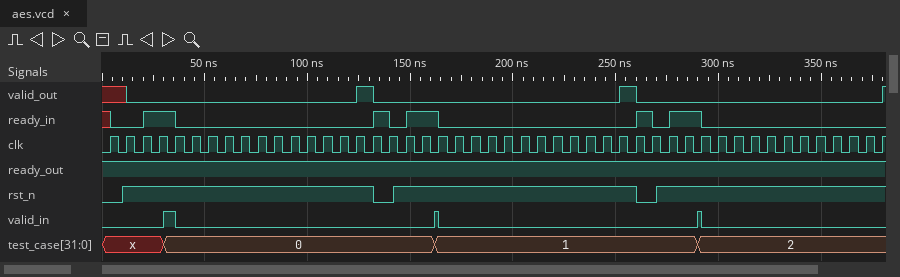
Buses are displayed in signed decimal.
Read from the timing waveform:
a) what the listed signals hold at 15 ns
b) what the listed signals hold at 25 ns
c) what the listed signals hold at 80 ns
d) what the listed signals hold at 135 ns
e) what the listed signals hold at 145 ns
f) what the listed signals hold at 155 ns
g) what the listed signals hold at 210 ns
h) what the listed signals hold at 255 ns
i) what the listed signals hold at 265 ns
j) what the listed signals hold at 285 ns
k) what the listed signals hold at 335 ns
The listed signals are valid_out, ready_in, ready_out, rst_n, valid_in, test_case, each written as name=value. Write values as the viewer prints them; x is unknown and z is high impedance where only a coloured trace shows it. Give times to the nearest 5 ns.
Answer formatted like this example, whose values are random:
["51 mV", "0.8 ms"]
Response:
["valid_out=0, ready_in=0, ready_out=1, rst_n=1, valid_in=0, test_case=x", "valid_out=0, ready_in=1, ready_out=1, rst_n=1, valid_in=0, test_case=x", "valid_out=0, ready_in=0, ready_out=1, rst_n=1, valid_in=0, test_case=0", "valid_out=0, ready_in=1, ready_out=1, rst_n=0, valid_in=0, test_case=0", "valid_out=0, ready_in=0, ready_out=1, rst_n=1, valid_in=0, test_case=0", "valid_out=0, ready_in=1, ready_out=1, rst_n=1, valid_in=0, test_case=0", "valid_out=0, ready_in=0, ready_out=1, rst_n=1, valid_in=0, test_case=1", "valid_out=1, ready_in=0, ready_out=1, rst_n=1, valid_in=0, test_case=1", "valid_out=0, ready_in=1, ready_out=1, rst_n=0, valid_in=0, test_case=1", "valid_out=0, ready_in=1, ready_out=1, rst_n=1, valid_in=0, test_case=1", "valid_out=0, ready_in=0, ready_out=1, rst_n=1, valid_in=0, test_case=2"]
